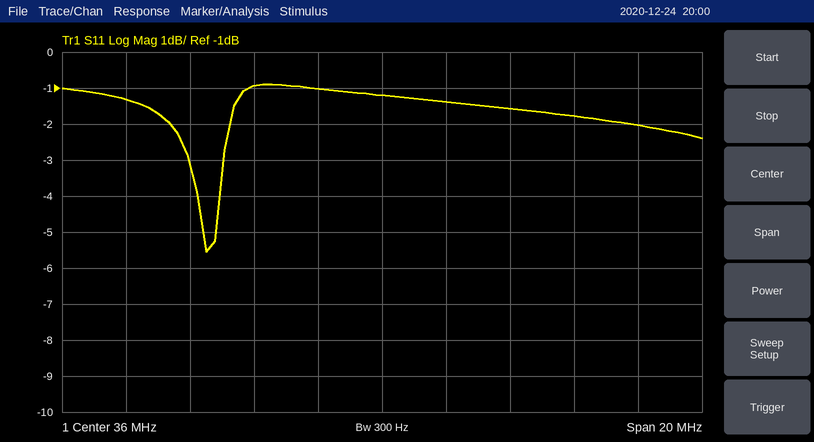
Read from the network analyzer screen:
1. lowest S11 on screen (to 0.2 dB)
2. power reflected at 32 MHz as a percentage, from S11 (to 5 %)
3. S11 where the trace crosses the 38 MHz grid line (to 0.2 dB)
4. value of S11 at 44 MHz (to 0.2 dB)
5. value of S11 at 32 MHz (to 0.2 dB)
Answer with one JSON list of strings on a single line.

["-5.6 dB", "80 %", "-1.4 dB", "-2.0 dB", "-1.0 dB"]
